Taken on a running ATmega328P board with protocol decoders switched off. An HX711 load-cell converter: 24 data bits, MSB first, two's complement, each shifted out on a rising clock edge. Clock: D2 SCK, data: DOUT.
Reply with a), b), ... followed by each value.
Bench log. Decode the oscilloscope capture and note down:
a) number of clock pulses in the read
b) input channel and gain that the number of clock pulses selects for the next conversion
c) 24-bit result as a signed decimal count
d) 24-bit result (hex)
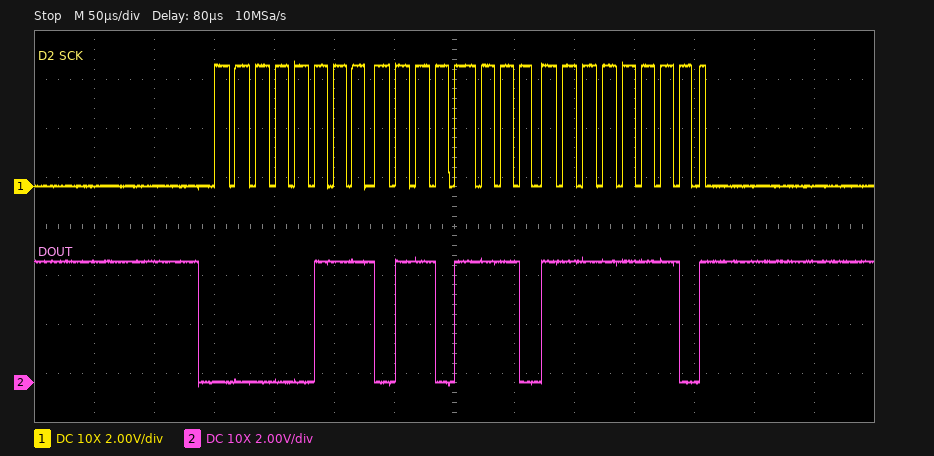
a) 25
b) channel A, gain 128
c) 487166
d) 0x076EFE
